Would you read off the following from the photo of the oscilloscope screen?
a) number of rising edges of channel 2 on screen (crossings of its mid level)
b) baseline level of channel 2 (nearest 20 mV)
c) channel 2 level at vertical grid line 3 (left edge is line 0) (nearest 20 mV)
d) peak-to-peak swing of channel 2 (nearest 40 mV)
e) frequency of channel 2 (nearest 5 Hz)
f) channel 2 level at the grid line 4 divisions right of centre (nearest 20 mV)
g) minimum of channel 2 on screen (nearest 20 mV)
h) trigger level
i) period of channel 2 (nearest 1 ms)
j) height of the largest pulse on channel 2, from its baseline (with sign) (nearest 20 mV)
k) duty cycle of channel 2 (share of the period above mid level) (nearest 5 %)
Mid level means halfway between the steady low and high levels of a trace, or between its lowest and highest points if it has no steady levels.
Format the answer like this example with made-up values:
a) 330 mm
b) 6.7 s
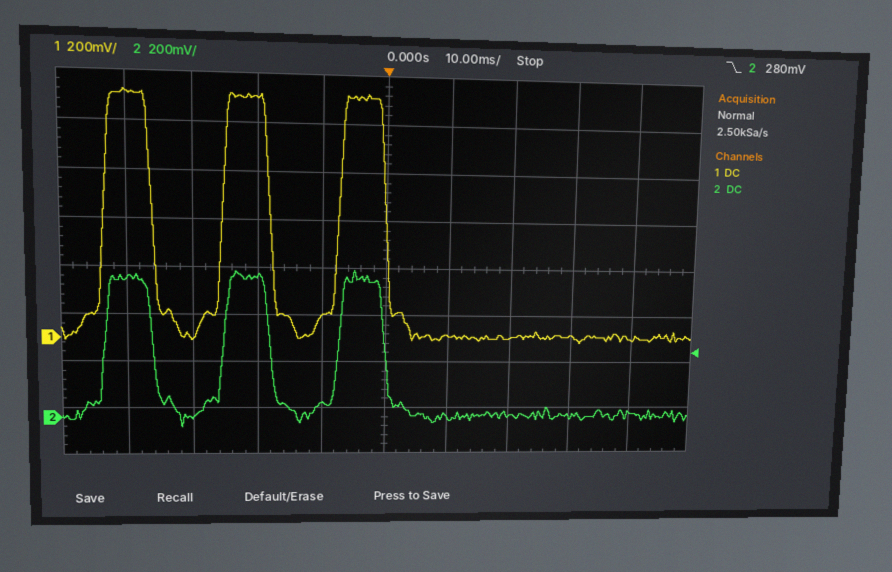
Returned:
a) 3
b) 0 mV
c) 600 mV
d) 680 mV
e) 55 Hz
f) 0 mV
g) -40 mV
h) 280 mV
i) 18 ms
j) +620 mV
k) 40 %
